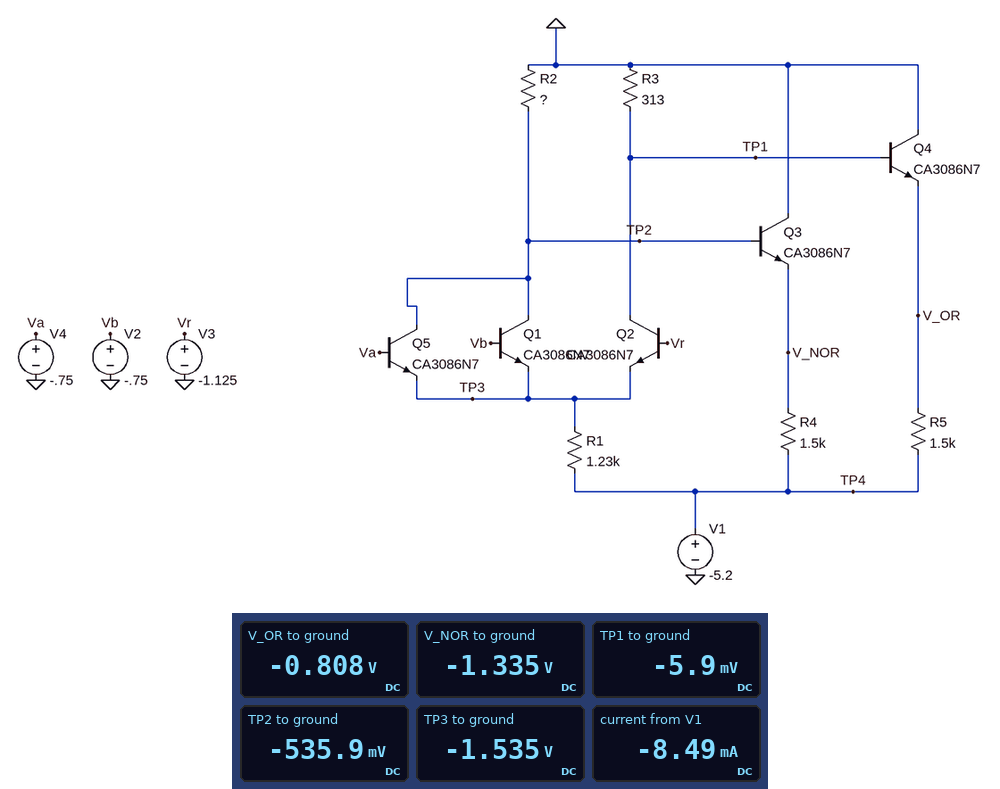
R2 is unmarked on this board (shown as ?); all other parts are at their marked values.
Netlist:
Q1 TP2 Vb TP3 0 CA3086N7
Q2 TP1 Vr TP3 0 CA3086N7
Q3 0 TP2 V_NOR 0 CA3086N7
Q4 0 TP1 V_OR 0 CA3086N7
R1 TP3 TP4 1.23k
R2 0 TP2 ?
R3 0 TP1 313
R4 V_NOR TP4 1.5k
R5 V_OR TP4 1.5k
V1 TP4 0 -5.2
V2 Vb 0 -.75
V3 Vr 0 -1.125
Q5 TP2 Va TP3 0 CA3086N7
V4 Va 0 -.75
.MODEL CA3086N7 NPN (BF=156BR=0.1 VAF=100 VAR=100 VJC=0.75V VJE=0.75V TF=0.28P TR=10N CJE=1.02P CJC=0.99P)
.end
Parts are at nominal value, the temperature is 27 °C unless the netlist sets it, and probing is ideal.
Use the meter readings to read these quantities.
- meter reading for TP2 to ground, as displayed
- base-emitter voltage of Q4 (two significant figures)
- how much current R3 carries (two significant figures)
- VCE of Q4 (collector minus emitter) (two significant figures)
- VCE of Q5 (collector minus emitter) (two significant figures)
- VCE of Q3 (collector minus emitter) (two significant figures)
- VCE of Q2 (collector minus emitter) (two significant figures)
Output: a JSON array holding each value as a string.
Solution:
["-535.9 mV", "800 mV", "19 µA", "810 mV", "1.0 V", "1.3 V", "1.5 V"]
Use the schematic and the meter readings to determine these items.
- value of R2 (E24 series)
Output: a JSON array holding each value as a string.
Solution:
["180 Ω"]
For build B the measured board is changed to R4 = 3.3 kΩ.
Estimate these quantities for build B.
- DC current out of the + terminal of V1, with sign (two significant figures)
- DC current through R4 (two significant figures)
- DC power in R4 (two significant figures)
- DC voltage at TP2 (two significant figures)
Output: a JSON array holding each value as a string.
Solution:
["-7.1 mA", "1.2 mA", "4.6 mW", "-530 mV"]
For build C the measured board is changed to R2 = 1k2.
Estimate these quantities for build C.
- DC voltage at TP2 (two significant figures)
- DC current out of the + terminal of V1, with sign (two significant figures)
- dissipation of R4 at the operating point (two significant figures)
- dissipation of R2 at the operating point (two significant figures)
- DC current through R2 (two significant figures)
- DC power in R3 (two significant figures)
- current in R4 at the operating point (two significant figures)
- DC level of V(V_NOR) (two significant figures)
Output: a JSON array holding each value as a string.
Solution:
["-1.5 V", "-7.8 mA", "5.6 mW", "1.9 mW", "1.3 mA", "110 nW", "1.9 mA", "-2.3 V"]
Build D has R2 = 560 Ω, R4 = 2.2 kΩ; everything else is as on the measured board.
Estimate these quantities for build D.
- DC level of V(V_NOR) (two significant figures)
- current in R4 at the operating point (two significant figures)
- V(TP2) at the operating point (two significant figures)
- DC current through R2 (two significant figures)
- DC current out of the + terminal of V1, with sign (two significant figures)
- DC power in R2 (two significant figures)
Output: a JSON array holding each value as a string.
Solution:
["-2.3 V", "1.3 mA", "-1.5 V", "2.6 mA", "-7.2 mA", "3.9 mW"]
